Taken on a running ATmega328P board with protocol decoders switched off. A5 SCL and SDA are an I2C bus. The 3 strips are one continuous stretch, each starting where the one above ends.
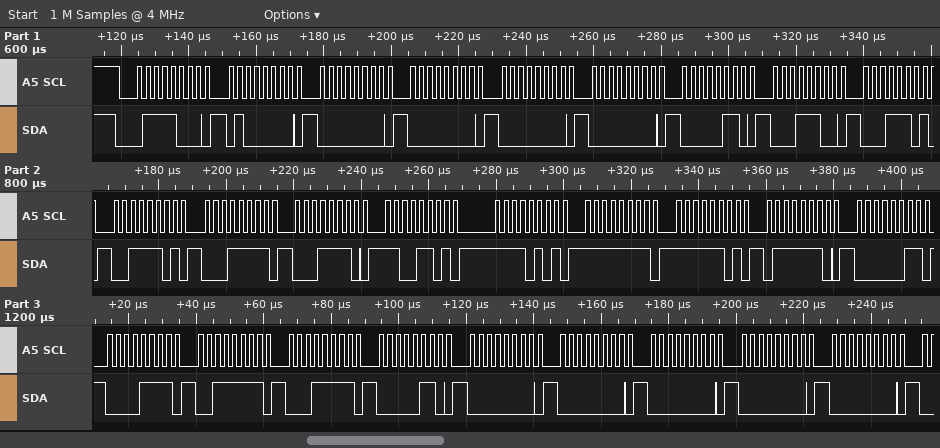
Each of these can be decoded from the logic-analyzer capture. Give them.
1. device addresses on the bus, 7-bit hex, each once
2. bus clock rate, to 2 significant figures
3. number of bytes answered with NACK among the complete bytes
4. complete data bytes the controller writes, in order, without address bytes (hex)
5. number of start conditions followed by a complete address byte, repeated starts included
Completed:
0x3C
400 kHz
0
40 00 00 00 00 06 1C 1D 3D 1F 1E CD F5 FF FD 7E 03 0F 3F 1F 06 00 00 00 00 00
1
